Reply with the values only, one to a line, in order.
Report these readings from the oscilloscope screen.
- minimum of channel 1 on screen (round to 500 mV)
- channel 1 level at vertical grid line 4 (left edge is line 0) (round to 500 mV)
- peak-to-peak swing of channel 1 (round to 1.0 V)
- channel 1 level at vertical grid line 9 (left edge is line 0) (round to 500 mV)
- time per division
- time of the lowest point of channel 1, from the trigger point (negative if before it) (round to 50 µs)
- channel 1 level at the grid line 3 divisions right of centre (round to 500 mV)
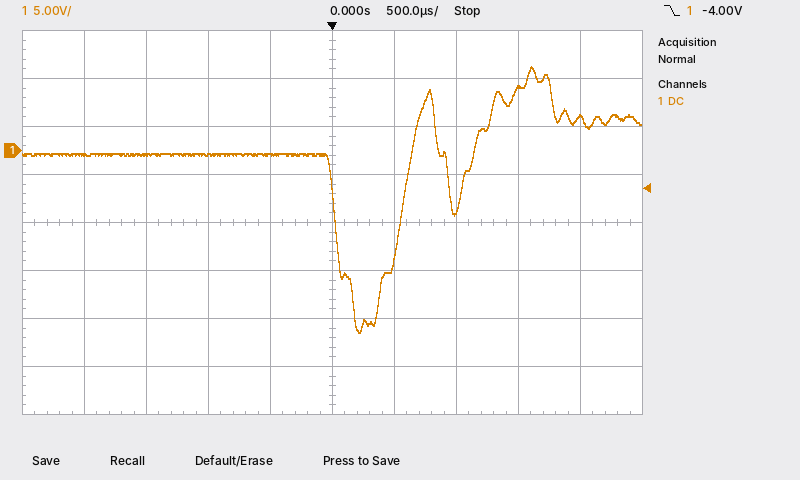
-19.0 V
-500 mV
28.0 V
3.5 V
500 µs
+200 µs
6.5 V
